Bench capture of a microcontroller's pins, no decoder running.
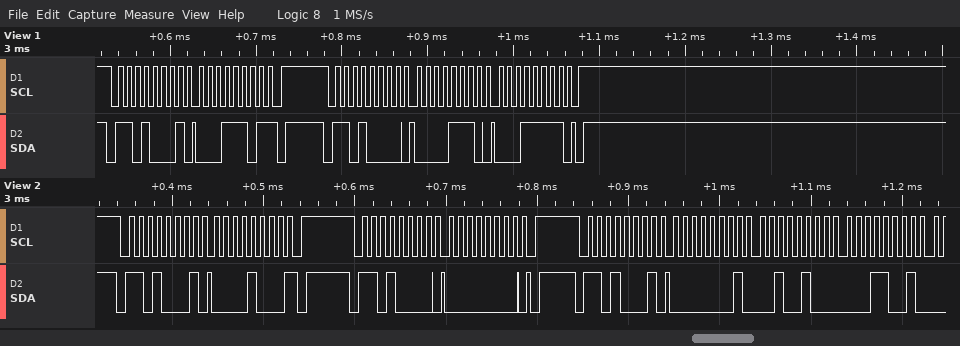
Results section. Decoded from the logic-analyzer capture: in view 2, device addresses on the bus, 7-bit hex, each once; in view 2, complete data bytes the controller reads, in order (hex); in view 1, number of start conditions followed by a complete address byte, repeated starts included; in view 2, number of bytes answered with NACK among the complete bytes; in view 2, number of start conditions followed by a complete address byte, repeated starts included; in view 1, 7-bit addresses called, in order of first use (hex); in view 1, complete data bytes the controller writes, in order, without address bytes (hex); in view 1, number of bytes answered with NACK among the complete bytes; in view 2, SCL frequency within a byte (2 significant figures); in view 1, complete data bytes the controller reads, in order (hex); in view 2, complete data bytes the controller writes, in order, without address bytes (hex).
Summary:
0x68
08 01 24 19
2
1
3
0x68
0E 1F
1
100 kHz
1D
00
